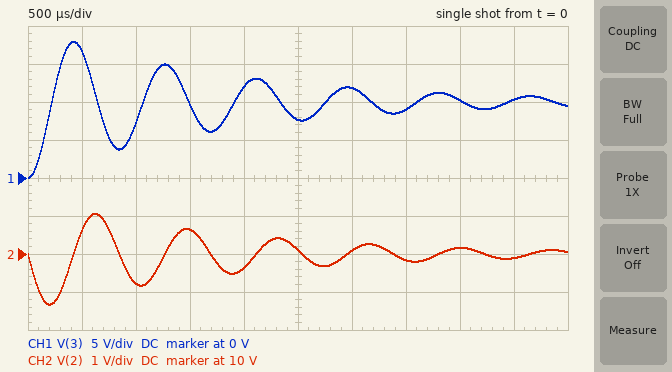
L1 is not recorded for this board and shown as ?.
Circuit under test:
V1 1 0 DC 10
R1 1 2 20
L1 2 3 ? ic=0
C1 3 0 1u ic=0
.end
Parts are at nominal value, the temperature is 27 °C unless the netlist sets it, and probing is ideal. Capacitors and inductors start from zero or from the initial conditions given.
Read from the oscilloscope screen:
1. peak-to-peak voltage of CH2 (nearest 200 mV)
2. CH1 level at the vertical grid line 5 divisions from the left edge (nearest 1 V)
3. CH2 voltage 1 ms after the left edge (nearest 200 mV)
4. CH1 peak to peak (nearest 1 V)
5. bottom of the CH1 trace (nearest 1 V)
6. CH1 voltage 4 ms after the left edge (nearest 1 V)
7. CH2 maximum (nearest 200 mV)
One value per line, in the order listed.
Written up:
2.4 V
8 V
9.2 V
18 V
0 V
10 V
11.0 V
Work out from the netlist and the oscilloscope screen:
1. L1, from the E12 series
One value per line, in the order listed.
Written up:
18 mH
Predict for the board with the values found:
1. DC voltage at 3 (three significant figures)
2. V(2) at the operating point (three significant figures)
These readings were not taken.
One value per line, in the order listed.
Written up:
10.0 V
10.0 V
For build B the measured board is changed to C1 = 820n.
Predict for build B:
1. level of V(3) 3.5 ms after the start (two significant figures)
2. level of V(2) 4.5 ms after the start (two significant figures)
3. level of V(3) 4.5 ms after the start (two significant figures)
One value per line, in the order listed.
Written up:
11 V
10 V
9.4 V
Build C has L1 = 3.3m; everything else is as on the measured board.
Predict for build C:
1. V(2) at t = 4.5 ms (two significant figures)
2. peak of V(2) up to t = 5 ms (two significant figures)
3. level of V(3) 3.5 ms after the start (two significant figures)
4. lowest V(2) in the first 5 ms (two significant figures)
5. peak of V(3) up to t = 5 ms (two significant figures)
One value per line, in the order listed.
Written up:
10 V
12 V
10 V
7.3 V
16 V
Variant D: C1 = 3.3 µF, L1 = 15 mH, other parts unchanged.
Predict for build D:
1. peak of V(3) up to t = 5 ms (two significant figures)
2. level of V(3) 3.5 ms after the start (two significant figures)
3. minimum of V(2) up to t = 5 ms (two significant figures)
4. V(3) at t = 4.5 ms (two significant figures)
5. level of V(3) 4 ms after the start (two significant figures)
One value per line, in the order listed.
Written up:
16 V
11 V
7.6 V
9.7 V
9.8 V
